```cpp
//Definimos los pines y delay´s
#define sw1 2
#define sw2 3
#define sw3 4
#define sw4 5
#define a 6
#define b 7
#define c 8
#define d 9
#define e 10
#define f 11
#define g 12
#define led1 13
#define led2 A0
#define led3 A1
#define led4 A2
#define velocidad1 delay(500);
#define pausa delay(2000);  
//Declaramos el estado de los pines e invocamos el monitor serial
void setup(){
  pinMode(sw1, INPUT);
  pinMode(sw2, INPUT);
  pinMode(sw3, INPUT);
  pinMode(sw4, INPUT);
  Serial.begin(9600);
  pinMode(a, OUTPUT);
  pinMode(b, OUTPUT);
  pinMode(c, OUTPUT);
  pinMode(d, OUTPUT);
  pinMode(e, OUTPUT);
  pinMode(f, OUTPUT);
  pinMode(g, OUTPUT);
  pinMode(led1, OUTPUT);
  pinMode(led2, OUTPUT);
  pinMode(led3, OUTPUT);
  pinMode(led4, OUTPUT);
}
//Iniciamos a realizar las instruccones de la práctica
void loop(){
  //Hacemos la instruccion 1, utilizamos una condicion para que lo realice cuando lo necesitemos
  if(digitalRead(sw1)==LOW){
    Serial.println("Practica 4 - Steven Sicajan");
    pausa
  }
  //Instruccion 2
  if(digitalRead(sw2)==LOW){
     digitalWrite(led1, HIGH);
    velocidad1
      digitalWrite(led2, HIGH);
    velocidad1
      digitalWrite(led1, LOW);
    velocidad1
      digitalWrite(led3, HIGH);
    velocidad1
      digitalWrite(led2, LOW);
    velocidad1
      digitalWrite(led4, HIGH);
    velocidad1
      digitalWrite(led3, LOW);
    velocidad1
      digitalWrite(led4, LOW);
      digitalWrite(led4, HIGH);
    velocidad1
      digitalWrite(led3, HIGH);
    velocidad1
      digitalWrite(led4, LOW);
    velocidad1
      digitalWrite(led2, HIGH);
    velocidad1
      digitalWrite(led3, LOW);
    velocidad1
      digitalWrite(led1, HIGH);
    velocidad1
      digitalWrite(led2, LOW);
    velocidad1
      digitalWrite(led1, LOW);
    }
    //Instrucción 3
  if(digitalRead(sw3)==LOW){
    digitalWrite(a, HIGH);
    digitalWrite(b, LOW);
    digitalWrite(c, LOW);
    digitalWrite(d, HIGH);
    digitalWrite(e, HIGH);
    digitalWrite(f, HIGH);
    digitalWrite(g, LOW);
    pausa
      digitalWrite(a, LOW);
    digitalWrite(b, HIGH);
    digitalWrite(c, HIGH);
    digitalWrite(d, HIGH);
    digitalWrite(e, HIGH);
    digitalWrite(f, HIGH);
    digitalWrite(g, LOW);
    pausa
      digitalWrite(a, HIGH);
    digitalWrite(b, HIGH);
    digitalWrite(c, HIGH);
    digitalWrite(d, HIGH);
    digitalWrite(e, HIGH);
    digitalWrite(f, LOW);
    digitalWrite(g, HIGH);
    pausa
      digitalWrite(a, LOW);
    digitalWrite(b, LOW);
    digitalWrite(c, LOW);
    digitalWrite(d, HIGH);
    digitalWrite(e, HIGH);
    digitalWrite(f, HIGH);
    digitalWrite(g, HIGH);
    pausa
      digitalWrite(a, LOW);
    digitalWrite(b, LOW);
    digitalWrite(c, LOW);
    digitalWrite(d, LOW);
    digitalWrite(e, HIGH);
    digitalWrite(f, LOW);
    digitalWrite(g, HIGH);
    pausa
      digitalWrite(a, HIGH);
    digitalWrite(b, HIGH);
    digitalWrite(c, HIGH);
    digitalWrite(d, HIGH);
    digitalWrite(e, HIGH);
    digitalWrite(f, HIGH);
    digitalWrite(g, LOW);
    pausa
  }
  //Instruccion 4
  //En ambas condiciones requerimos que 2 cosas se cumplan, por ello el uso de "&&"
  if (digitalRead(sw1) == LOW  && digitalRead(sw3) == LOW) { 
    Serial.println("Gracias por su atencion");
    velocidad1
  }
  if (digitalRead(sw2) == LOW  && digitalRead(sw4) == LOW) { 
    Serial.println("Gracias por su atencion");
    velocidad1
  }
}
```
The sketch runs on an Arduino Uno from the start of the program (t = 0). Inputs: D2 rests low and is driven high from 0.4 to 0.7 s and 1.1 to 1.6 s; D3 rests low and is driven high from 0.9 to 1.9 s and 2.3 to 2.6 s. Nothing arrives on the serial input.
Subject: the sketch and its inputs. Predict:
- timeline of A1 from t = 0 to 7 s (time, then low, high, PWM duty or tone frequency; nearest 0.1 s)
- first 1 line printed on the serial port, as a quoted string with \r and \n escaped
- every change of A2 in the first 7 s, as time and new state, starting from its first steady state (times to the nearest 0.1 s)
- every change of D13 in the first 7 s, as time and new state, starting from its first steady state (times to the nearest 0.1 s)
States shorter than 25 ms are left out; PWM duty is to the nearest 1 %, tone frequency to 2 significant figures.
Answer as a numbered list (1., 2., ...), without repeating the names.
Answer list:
1. 0 s low; 3.5 s high; 5 s low; 6 s high
2. "Practica 4 - Steven Sicajan\r\n"
3. 0 s low; 4.5 s high; 6.5 s low
4. 0 s low; 2 s high; 3 s low
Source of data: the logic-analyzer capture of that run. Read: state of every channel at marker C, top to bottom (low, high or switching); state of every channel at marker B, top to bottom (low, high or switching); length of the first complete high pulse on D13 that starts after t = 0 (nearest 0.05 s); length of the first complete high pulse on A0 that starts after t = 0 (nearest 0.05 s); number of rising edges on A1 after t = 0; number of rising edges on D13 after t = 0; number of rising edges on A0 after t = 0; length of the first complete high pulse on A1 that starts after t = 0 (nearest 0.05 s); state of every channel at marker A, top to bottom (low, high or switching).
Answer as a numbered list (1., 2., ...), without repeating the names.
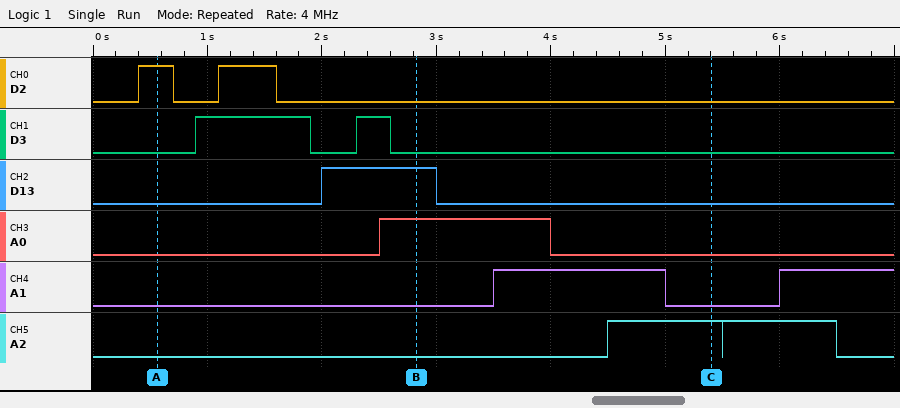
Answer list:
1. D2 low, D3 low, D13 low, A0 low, A1 low, A2 high
2. D2 low, D3 low, D13 high, A0 high, A1 low, A2 low
3. 1.00 s
4. 1.50 s
5. 2
6. 1
7. 1
8. 1.50 s
9. D2 high, D3 low, D13 low, A0 low, A1 low, A2 low
